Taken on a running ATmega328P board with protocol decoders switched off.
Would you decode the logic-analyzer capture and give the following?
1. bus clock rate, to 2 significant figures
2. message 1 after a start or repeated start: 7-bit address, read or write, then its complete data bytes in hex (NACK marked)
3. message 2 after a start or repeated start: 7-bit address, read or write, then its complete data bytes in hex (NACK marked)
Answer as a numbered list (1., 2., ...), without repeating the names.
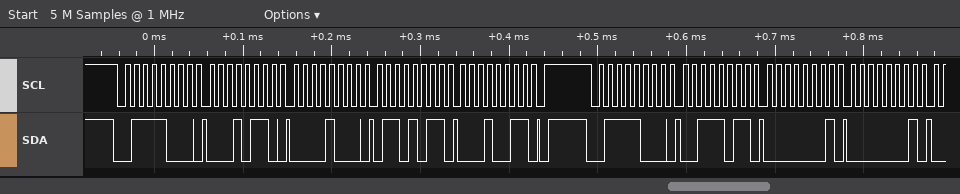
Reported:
1. 100 kHz
2. 0x3C write: 16 08 6B 13
3. 0x3C write: 3B 01 01
